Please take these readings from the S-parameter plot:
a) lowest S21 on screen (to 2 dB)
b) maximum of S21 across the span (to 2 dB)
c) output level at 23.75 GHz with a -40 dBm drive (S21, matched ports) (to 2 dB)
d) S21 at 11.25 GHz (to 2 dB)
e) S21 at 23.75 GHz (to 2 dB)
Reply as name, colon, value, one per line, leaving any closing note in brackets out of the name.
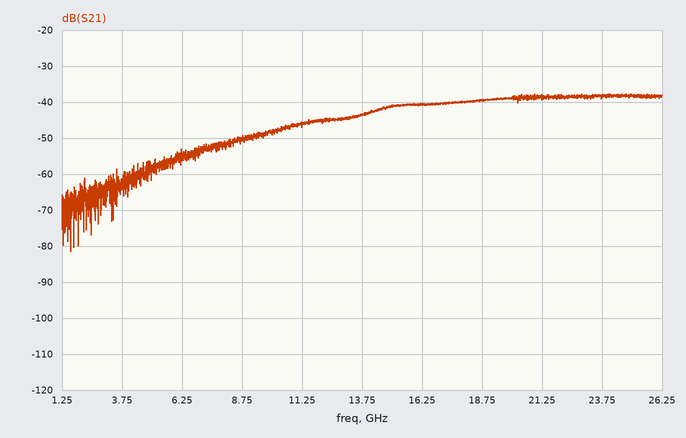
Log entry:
lowest S21 on screen: -82 dB
maximum of S21 across the span: -38 dB
output level at 23.75 GHz with a -40 dBm drive (S21, matched ports): -78 dBm
S21 at 11.25 GHz: -46 dB
S21 at 23.75 GHz: -38 dB
